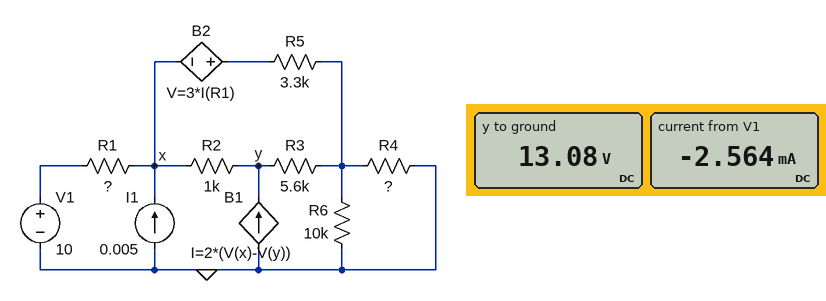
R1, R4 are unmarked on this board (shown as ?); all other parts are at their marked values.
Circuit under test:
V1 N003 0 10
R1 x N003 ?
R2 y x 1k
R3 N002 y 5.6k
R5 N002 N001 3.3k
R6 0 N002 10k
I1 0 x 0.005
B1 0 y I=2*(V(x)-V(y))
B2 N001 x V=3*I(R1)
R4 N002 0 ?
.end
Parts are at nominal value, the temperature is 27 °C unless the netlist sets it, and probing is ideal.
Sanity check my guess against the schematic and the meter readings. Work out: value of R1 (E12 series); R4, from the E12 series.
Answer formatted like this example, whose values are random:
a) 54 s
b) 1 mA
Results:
a) 1.2 kΩ
b) 1.5 kΩ
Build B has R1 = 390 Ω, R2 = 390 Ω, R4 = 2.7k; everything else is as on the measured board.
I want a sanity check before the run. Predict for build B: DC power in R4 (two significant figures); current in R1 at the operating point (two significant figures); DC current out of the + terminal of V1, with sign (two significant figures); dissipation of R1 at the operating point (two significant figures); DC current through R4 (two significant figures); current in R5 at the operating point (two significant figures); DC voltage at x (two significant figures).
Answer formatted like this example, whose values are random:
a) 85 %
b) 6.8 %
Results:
a) 12 mW
b) 3.3 mA
c) -3.3 mA
d) 4.3 mW
e) 2.1 mA
f) 1.7 mA
g) 11 V
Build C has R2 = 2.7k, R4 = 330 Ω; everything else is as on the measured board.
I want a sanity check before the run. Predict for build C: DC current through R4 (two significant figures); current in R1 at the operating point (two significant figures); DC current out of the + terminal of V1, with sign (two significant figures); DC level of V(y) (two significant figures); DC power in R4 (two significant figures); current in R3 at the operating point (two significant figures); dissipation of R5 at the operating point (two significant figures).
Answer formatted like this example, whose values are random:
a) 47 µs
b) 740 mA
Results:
a) 4.9 mA
b) 1.8 mA
c) -1.8 mA
d) 12 V
e) 8.0 mW
f) 1.9 mA
g) 34 mW
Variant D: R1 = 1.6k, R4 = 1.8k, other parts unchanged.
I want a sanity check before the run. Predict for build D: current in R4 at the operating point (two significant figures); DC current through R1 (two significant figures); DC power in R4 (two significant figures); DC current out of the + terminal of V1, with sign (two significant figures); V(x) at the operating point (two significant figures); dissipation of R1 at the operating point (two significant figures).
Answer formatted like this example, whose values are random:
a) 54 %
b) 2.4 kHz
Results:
a) 3.3 mA
b) 2.5 mA
c) 20 mW
d) -2.5 mA
e) 14 V
f) 10 mW
